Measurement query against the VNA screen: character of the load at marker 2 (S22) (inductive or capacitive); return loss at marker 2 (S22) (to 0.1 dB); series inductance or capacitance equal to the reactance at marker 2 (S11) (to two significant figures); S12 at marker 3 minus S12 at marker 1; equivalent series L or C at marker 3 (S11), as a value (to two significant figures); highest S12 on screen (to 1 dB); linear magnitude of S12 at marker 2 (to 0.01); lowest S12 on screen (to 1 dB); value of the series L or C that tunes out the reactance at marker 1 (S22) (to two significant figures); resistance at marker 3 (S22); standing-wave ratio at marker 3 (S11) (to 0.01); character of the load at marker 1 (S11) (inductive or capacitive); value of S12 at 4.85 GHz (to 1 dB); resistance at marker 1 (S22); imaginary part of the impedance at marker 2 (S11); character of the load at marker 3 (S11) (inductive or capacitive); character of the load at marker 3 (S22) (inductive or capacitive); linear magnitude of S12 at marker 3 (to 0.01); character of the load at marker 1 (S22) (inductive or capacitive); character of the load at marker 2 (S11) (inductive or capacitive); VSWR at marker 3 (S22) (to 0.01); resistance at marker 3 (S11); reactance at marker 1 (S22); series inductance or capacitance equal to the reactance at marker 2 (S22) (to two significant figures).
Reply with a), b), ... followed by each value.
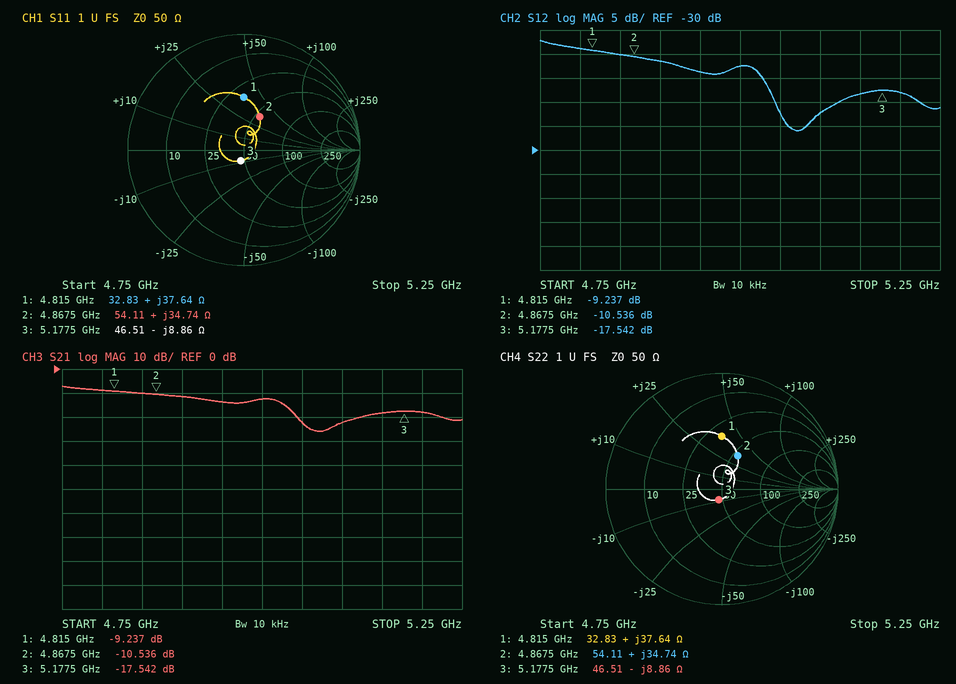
a) inductive
b) 9.9 dB
c) 1.1 nH
d) -8.305 dB
e) 3.5 pF
f) -7 dB
g) 0.30
h) -26 dB
i) 880 fF
j) 46.51 Ω
k) 1.22
l) inductive
m) -10 dB
n) 32.83 Ω
o) +34.74 Ω
p) capacitive
q) capacitive
r) 0.13
s) inductive
t) inductive
u) 1.22
v) 46.51 Ω
w) +37.64 Ω
x) 1.1 nH
